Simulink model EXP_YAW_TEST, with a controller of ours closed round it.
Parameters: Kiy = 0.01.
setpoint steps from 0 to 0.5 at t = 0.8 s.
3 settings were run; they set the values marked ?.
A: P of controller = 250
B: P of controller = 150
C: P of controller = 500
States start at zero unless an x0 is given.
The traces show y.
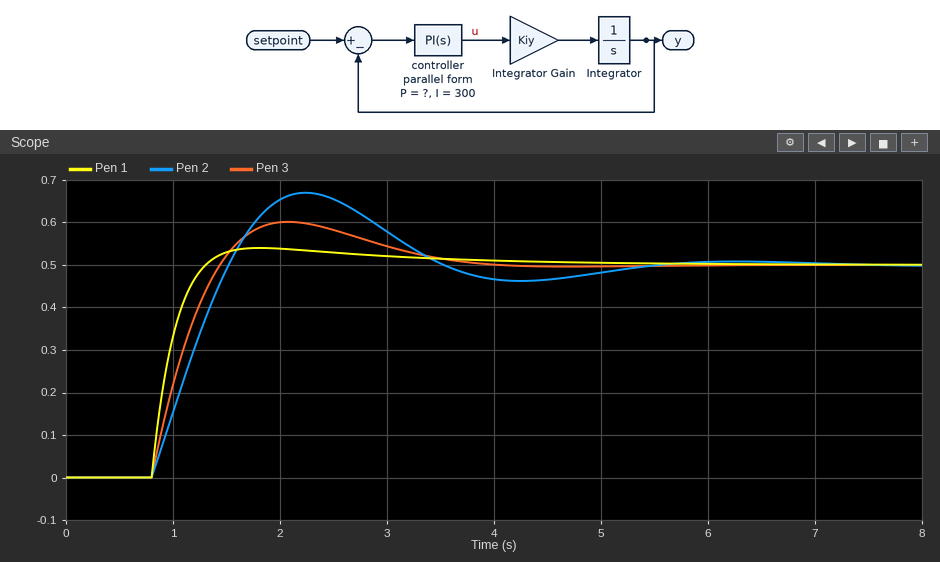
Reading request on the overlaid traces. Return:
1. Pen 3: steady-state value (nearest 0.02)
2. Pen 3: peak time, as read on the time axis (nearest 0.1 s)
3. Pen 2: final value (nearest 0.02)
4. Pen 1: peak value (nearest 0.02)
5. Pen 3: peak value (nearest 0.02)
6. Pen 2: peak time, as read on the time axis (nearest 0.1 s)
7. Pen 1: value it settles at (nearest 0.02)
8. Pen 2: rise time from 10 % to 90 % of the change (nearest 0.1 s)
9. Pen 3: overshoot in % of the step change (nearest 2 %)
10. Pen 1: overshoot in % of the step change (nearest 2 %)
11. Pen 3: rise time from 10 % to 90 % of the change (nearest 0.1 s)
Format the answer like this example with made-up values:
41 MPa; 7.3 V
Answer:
0.50; 2.1 s; 0.50; 0.54; 0.60; 2.2 s; 0.50; 0.6 s; 20 %; 8 %; 0.5 s
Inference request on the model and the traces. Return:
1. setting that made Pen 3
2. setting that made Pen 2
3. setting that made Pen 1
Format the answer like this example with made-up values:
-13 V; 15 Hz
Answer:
A; B; C
